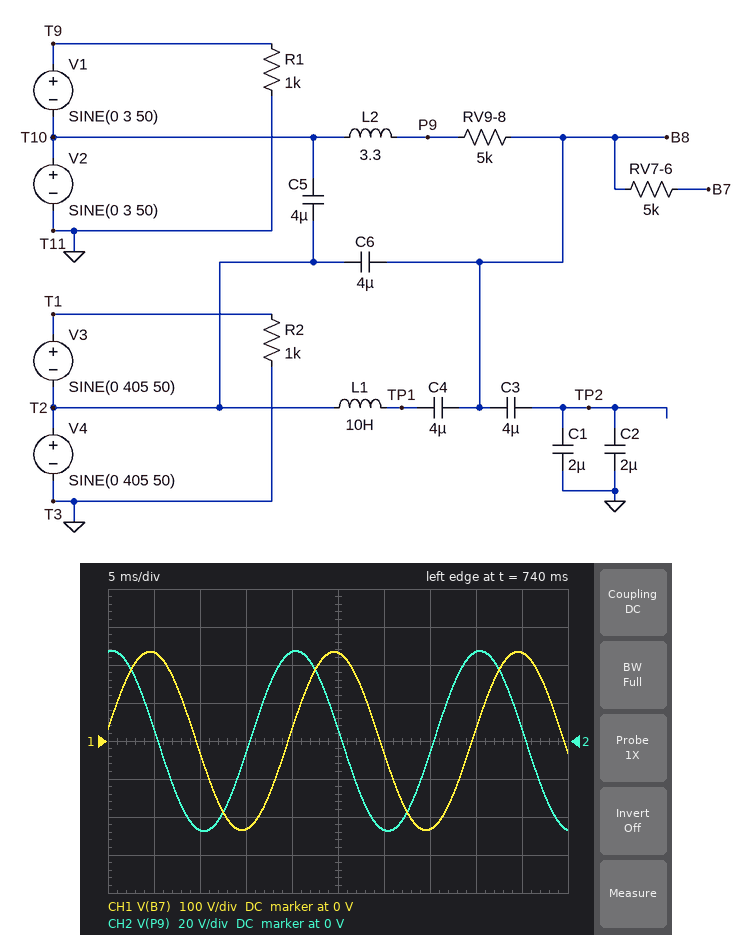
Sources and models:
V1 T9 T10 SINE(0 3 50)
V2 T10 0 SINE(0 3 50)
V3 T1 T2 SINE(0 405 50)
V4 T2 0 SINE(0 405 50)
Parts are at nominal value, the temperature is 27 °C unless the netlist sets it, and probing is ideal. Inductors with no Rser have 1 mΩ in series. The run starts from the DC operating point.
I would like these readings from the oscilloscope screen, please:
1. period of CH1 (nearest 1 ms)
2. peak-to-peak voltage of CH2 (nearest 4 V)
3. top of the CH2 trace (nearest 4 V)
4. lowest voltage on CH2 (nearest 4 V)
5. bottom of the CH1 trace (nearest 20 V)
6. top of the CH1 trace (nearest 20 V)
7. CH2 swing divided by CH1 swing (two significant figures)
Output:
20 ms
96 V
48 V
-48 V
-240 V
240 V
0.20
